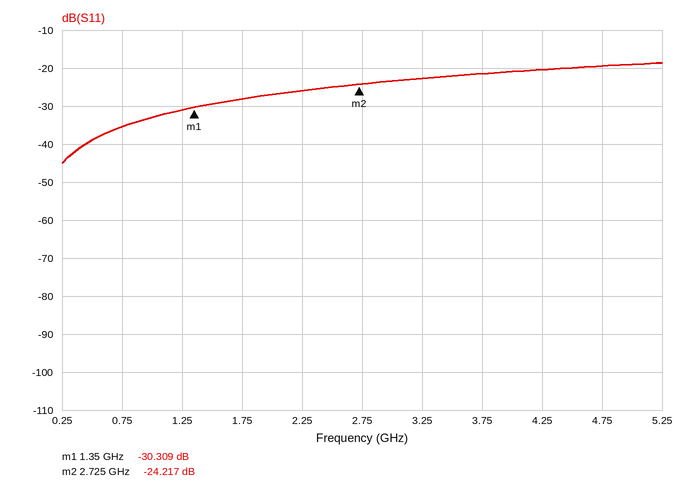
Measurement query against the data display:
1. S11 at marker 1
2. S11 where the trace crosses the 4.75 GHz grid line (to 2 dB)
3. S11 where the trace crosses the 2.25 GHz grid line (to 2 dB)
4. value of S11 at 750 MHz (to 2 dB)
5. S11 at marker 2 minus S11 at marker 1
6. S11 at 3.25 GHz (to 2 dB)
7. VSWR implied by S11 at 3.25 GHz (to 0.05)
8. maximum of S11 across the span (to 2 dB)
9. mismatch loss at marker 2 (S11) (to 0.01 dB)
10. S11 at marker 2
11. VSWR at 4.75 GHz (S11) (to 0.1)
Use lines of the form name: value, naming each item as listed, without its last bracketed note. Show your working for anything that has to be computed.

S11 at marker 1: -30.309 dB
S11 where the trace crosses the 4.75 GHz grid line: -20 dB
S11 where the trace crosses the 2.25 GHz grid line: -26 dB
value of S11 at 750 MHz: -36 dB
S11 at marker 2 minus S11 at marker 1: -24.217 − (-30.309) = 6.092 dB
S11 at 3.25 GHz: -22 dB
VSWR implied by S11 at 3.25 GHz: |Γ| = 10^(-22/20) = 0.0794; VSWR = (1 + 0.0794)/(1 − 0.0794) ≈ 1.17, so 1.15 to the nearest 0.05
maximum of S11 across the span: -18 dB
mismatch loss at marker 2 (S11): −10 log10(1 − 10^(-24.217/10)) ≈ 0.02 dB
S11 at marker 2: -24.217 dB
VSWR at 4.75 GHz (S11): |Γ| = 10^(-20/20) = 0.1000; VSWR = (1 + 0.1000)/(1 − 0.1000) ≈ 1.2
